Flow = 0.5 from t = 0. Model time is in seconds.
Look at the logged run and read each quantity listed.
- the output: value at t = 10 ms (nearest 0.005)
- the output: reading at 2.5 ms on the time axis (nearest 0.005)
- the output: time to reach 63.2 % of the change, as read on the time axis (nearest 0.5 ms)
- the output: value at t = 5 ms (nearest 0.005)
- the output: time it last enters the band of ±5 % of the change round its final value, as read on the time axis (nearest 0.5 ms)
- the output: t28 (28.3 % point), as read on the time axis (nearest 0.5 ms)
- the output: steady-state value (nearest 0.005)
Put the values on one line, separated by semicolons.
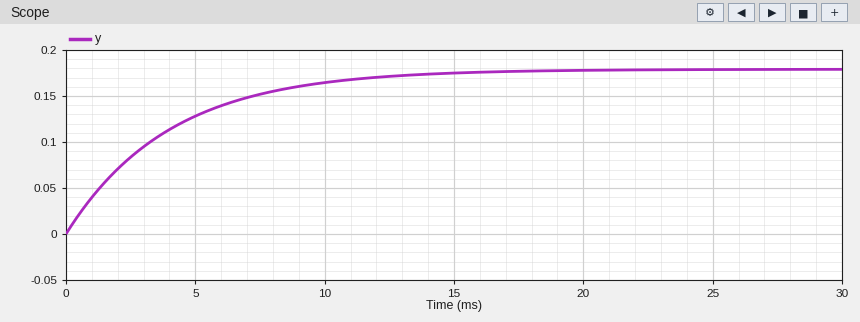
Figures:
0.165; 0.085; 4.0 ms; 0.130; 12.0 ms; 1.5 ms; 0.180
